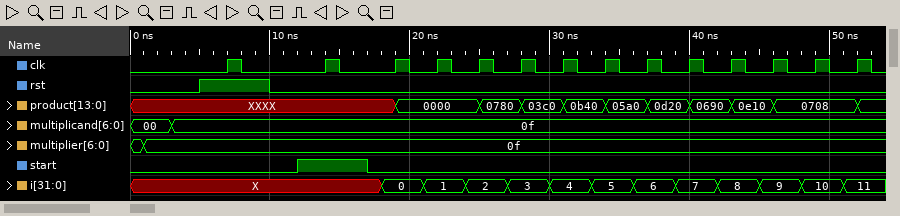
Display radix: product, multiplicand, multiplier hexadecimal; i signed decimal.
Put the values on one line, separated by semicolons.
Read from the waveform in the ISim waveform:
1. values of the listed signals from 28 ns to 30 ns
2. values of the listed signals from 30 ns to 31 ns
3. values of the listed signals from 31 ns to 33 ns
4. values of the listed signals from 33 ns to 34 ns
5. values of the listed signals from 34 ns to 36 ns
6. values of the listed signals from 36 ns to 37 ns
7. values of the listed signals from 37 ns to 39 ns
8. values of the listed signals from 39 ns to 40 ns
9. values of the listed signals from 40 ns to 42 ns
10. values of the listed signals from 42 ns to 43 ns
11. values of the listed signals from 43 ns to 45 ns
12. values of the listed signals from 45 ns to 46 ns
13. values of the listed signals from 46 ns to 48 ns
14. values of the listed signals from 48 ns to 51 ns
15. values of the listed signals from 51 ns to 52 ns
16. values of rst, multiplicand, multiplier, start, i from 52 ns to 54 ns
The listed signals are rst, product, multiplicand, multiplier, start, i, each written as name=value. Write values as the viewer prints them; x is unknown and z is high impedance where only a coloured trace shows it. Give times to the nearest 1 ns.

rst=0, product=03c0, multiplicand=0f, multiplier=0f, start=0, i=3; rst=0, product=03c0, multiplicand=0f, multiplier=0f, start=0, i=4; rst=0, product=0b40, multiplicand=0f, multiplier=0f, start=0, i=4; rst=0, product=0b40, multiplicand=0f, multiplier=0f, start=0, i=5; rst=0, product=05a0, multiplicand=0f, multiplier=0f, start=0, i=5; rst=0, product=05a0, multiplicand=0f, multiplier=0f, start=0, i=6; rst=0, product=0d20, multiplicand=0f, multiplier=0f, start=0, i=6; rst=0, product=0d20, multiplicand=0f, multiplier=0f, start=0, i=7; rst=0, product=0690, multiplicand=0f, multiplier=0f, start=0, i=7; rst=0, product=0690, multiplicand=0f, multiplier=0f, start=0, i=8; rst=0, product=0e10, multiplicand=0f, multiplier=0f, start=0, i=8; rst=0, product=0e10, multiplicand=0f, multiplier=0f, start=0, i=9; rst=0, product=0708, multiplicand=0f, multiplier=0f, start=0, i=9; rst=0, product=0708, multiplicand=0f, multiplier=0f, start=0, i=10; rst=0, product=0708, multiplicand=0f, multiplier=0f, start=0, i=11; rst=0, multiplicand=0f, multiplier=0f, start=0, i=11
